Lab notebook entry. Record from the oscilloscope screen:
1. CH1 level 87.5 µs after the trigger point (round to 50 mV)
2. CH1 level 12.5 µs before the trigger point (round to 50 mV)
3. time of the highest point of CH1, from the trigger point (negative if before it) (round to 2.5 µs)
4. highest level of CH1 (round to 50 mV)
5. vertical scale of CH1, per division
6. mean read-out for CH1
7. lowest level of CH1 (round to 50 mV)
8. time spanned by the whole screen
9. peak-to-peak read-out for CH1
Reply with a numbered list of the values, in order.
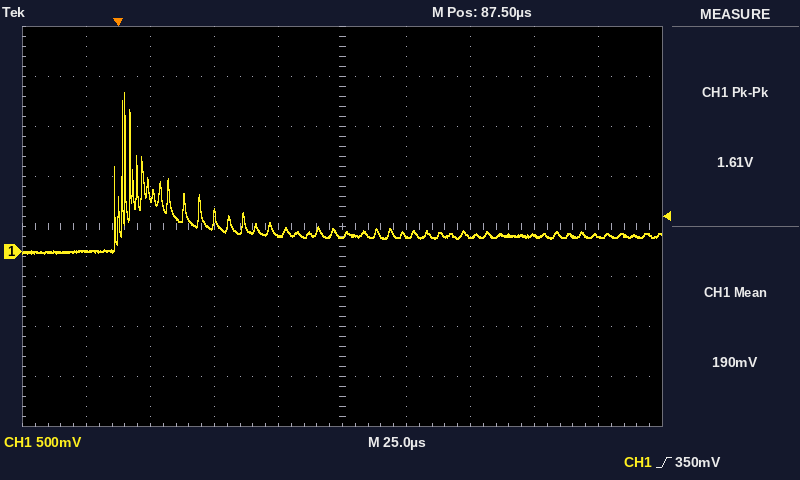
1. 150 mV
2. 0 mV
3. +2.5 µs
4. 1.60 V
5. 500 mV
6. 190 mV
7. 0 mV
8. 250 µs
9. 1.61 V
